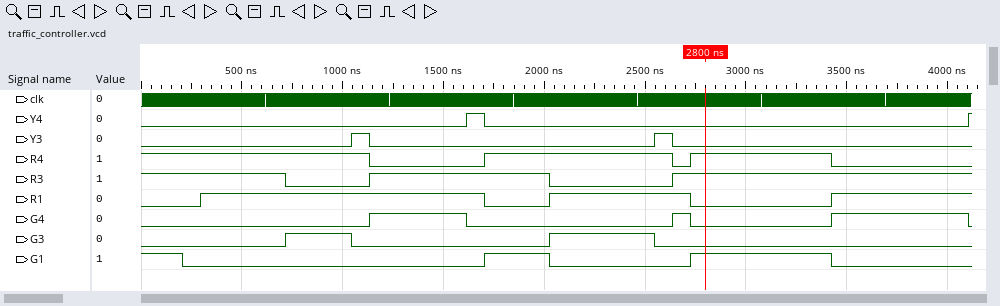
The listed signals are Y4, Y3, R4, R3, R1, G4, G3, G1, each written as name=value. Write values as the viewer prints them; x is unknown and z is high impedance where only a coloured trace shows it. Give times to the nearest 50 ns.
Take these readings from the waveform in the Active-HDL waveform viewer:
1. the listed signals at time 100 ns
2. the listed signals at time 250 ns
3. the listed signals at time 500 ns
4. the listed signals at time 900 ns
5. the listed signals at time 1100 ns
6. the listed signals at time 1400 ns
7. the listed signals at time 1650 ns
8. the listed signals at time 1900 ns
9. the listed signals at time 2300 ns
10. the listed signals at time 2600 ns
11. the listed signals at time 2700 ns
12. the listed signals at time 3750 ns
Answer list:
Y4=0, Y3=0, R4=1, R3=1, R1=0, G4=0, G3=0, G1=1
Y4=0, Y3=0, R4=1, R3=1, R1=0, G4=0, G3=0, G1=0
Y4=0, Y3=0, R4=1, R3=1, R1=1, G4=0, G3=0, G1=0
Y4=0, Y3=0, R4=1, R3=0, R1=1, G4=0, G3=1, G1=0
Y4=0, Y3=1, R4=1, R3=0, R1=1, G4=0, G3=0, G1=0
Y4=0, Y3=0, R4=0, R3=1, R1=1, G4=1, G3=0, G1=0
Y4=1, Y3=0, R4=0, R3=1, R1=1, G4=0, G3=0, G1=0
Y4=0, Y3=0, R4=1, R3=1, R1=0, G4=0, G3=0, G1=1
Y4=0, Y3=0, R4=1, R3=0, R1=1, G4=0, G3=1, G1=0
Y4=0, Y3=1, R4=1, R3=0, R1=1, G4=0, G3=0, G1=0
Y4=0, Y3=0, R4=0, R3=1, R1=1, G4=1, G3=0, G1=0
Y4=0, Y3=0, R4=0, R3=1, R1=1, G4=1, G3=0, G1=0
